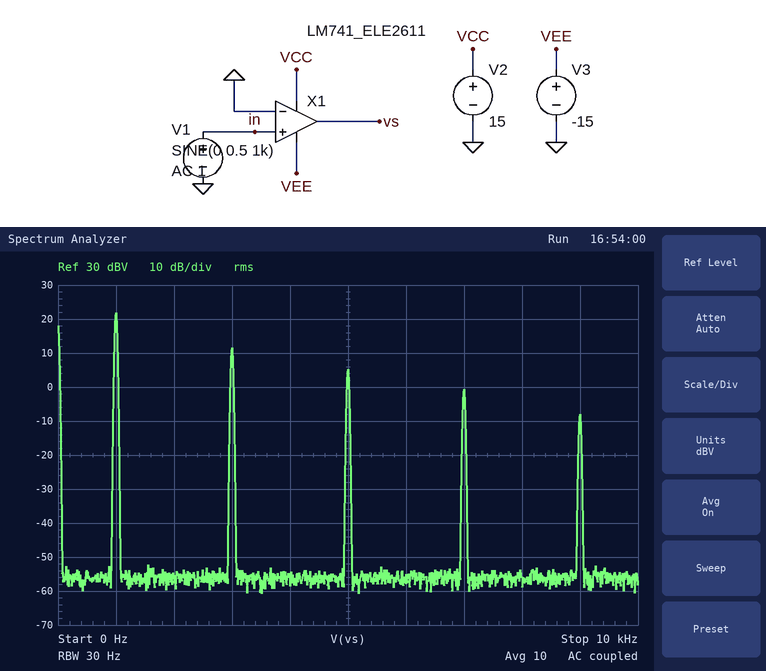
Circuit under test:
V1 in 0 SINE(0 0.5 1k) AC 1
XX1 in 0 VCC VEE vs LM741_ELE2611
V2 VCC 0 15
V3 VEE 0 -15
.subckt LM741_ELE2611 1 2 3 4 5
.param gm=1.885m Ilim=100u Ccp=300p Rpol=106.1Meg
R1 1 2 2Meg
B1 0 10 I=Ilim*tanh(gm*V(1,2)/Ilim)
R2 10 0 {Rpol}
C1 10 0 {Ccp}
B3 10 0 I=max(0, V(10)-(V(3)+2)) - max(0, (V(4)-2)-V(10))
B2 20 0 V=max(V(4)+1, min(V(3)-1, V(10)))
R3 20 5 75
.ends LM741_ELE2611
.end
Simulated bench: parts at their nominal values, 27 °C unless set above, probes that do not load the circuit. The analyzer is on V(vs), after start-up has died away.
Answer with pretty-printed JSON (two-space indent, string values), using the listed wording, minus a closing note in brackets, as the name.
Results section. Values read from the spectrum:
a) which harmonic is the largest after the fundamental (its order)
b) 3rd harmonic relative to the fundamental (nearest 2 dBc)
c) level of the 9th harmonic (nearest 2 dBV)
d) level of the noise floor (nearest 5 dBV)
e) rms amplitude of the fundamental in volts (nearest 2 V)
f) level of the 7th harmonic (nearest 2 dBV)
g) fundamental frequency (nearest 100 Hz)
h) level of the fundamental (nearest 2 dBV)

{
  "which harmonic is the largest after the fundamental": "3",
  "3rd harmonic relative to the fundamental": "-10 dBc",
  "level of the 9th harmonic": "-8 dBV",
  "level of the noise floor": "-55 dBV",
  "rms amplitude of the fundamental in volts": "12 V",
  "level of the 7th harmonic": "0 dBV",
  "fundamental frequency": "1.0 kHz",
  "level of the fundamental": "22 dBV"
}
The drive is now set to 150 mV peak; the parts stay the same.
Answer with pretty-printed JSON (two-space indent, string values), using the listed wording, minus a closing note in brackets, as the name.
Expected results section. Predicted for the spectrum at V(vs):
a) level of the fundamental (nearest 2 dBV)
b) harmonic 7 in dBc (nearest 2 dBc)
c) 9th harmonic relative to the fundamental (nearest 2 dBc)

{
  "level of the fundamental": "22 dBV",
  "harmonic 7 in dBc": "-24 dBc",
  "9th harmonic relative to the fundamental": "-34 dBc"
}
